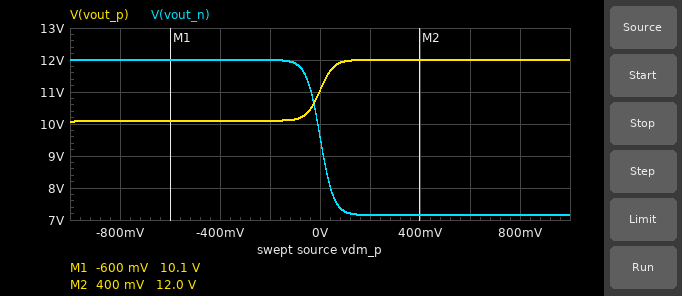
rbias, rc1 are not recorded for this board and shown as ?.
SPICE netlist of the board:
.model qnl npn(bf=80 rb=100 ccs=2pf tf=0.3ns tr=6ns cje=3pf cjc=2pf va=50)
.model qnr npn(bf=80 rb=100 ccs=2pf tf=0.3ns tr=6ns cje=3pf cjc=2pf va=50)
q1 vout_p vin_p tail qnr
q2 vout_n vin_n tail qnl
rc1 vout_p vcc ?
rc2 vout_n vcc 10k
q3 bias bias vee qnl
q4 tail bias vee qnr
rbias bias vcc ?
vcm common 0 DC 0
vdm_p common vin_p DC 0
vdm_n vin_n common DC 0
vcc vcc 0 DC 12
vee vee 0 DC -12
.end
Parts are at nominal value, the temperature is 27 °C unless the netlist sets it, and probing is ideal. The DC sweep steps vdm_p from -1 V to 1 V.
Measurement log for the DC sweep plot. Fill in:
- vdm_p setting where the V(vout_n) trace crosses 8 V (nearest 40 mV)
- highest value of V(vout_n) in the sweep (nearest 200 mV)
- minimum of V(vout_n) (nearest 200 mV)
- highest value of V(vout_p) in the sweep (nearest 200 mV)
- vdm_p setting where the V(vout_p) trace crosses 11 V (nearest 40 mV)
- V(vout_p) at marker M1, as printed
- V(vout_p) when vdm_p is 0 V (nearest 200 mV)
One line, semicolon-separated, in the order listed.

40 mV; 12.0 V; 7.2 V; 12.0 V; 0 V; 10.1 V; 11.0 V
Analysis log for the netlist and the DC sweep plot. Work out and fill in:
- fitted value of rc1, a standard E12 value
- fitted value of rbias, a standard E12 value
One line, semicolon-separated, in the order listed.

3.9 kΩ; 56 kΩ
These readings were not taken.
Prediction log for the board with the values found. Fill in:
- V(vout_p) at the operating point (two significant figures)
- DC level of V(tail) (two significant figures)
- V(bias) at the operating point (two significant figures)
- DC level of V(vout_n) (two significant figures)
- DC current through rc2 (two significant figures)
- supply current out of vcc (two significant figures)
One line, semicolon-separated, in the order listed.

11 V; -730 mV; -11 V; 9.6 V; 240 µA; 900 µA
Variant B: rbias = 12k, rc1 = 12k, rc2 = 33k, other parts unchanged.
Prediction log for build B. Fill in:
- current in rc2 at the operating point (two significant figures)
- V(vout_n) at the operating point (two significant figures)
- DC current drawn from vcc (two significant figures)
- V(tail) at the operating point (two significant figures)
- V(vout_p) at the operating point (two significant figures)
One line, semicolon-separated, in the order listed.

390 µA; -800 mV; 3.4 mA; -830 mV; -780 mV
